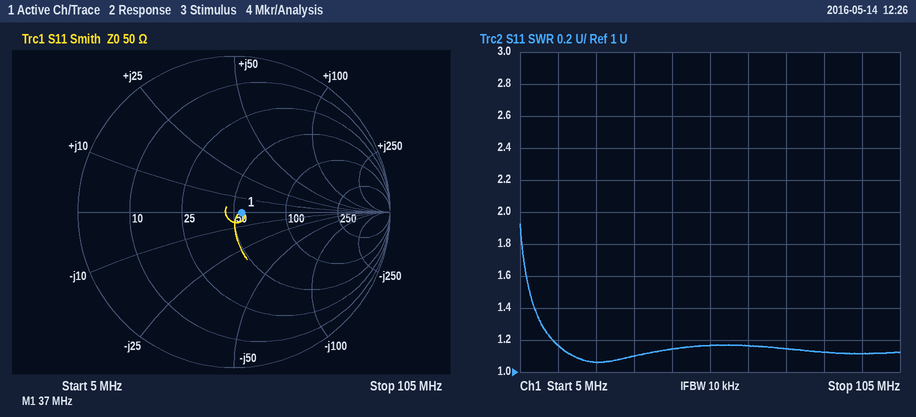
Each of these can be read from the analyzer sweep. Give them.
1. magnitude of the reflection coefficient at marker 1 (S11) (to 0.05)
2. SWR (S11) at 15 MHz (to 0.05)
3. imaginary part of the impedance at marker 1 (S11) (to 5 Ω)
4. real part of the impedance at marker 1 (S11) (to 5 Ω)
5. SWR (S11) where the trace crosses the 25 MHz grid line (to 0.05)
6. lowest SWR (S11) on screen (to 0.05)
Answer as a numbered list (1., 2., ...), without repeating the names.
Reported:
1. 0.05
2. 1.15
3. 0 Ω
4. 55 Ω
5. 1.05
6. 1.05
